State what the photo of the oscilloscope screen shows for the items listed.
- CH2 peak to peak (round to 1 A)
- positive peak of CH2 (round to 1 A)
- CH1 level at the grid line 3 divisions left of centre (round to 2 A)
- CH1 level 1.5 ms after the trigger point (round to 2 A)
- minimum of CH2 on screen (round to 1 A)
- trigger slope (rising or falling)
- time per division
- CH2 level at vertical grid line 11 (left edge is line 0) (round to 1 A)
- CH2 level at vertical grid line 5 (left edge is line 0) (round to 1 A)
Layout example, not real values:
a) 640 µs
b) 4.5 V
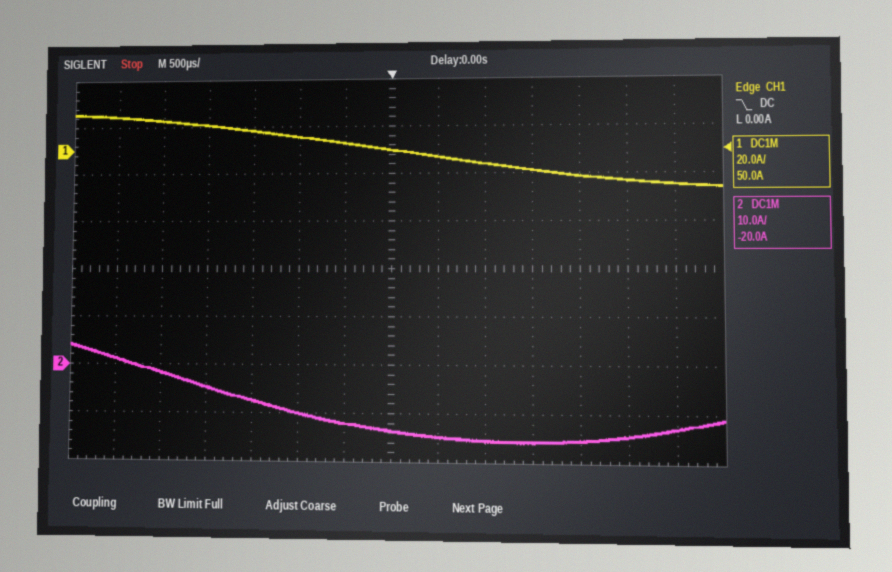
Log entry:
a) 20 A
b) 4 A
c) 8 A
d) -8 A
e) -16 A
f) falling
g) 500 µs
h) -15 A
i) -10 A
